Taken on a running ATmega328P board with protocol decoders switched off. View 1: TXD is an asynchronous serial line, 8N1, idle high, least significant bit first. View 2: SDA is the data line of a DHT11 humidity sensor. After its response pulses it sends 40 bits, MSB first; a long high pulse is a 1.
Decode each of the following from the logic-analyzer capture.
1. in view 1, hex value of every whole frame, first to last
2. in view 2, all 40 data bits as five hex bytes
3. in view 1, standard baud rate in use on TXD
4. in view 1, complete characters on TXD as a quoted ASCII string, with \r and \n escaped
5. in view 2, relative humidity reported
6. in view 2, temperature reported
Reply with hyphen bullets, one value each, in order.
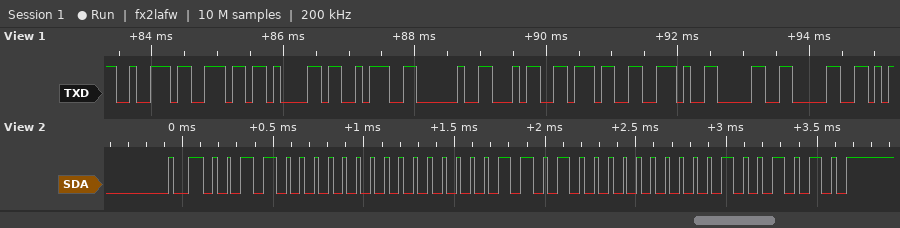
- 72 6E 61 3A 20 34 37 2E 30 30
- 30 00 1A 00 4A
- 9600 baud
- "rna: 47.00"
- 48 %
- 26.0 °C
